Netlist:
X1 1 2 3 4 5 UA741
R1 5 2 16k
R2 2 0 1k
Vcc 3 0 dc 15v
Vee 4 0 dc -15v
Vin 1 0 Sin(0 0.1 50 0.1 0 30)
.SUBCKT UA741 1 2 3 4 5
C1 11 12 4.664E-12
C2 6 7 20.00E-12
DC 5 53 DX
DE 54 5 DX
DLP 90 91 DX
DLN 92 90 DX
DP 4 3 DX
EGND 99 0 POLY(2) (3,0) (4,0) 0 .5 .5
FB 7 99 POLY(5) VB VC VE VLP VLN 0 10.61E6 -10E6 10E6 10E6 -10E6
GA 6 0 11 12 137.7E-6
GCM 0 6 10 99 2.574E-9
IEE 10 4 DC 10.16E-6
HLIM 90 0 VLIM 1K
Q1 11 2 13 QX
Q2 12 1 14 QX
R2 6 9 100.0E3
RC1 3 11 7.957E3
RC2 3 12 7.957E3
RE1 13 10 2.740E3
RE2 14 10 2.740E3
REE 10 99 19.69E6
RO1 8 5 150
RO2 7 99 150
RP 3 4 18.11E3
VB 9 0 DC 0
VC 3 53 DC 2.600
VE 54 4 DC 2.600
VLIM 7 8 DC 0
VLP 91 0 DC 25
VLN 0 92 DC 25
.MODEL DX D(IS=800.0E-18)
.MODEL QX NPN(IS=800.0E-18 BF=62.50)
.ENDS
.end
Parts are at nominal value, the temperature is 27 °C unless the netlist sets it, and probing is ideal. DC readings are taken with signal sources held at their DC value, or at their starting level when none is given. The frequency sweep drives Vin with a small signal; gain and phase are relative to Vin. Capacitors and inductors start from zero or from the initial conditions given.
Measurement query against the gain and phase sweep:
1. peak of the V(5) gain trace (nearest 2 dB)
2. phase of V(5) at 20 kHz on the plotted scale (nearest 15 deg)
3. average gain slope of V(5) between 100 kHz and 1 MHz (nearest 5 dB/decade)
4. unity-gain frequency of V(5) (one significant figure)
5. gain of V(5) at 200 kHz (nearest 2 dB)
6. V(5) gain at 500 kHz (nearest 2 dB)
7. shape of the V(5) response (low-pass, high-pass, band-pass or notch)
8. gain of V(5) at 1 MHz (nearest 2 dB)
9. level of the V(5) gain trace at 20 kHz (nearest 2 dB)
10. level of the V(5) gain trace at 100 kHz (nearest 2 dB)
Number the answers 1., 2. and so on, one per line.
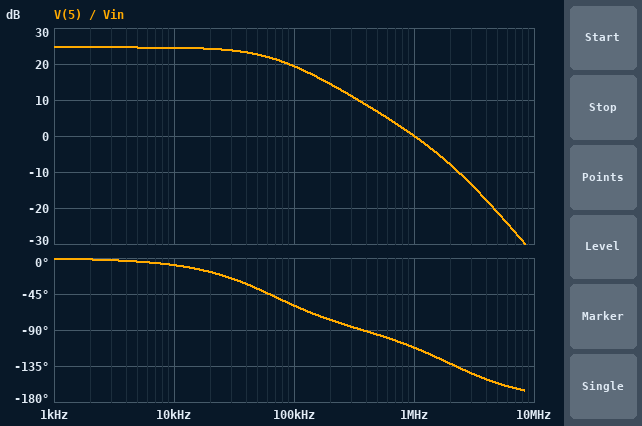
1. 24 dB
2. -15 deg
3. -20 dB/decade
4. 1 MHz
5. 14 dB
6. 6 dB
7. low-pass
8. 0 dB
9. 24 dB
10. 20 dB
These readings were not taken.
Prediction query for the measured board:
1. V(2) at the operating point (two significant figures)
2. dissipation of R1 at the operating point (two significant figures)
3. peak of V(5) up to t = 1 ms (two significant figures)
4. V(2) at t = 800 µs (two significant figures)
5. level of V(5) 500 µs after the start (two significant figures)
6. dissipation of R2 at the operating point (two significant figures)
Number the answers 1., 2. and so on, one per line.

1. 50 mV
2. 40 µW
3. 850 mV
4. 50 mV
5. 850 mV
6. 2.5 µW
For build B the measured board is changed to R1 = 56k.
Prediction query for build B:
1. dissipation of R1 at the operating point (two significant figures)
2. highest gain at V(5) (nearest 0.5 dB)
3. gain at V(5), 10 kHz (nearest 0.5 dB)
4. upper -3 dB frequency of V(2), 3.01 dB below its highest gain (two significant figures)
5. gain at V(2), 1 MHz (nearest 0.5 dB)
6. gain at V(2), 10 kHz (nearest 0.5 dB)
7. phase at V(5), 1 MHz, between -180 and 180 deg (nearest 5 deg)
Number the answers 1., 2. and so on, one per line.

1. 140 µW
2. 35.0 dB
3. 34.0 dB
4. 19 kHz
5. -35.5 dB
6. -1.0 dB
7. -115 deg
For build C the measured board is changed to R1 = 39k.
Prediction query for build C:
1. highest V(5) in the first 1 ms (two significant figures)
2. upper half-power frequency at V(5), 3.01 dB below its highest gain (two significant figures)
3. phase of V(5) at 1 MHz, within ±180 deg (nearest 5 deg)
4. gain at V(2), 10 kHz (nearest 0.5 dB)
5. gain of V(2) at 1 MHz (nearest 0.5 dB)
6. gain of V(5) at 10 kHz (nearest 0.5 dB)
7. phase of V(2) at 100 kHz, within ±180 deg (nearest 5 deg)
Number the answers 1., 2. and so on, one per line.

1. 2.0 V
2. 28 kHz
3. -115 deg
4. -0.5 dB
5. -32.0 dB
6. 31.5 dB
7. -75 deg
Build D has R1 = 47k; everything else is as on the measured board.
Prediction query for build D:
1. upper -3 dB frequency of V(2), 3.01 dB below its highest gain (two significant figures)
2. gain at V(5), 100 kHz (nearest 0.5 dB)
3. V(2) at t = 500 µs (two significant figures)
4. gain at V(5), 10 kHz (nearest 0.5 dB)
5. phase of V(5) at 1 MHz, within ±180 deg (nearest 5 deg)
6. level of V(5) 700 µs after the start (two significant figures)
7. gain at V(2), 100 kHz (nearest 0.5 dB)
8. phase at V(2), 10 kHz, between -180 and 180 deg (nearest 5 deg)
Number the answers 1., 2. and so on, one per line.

1. 23 kHz
2. 20.5 dB
3. 50 mV
4. 33.0 dB
5. -115 deg
6. 2.4 V
7. -13.0 dB
8. -25 deg
